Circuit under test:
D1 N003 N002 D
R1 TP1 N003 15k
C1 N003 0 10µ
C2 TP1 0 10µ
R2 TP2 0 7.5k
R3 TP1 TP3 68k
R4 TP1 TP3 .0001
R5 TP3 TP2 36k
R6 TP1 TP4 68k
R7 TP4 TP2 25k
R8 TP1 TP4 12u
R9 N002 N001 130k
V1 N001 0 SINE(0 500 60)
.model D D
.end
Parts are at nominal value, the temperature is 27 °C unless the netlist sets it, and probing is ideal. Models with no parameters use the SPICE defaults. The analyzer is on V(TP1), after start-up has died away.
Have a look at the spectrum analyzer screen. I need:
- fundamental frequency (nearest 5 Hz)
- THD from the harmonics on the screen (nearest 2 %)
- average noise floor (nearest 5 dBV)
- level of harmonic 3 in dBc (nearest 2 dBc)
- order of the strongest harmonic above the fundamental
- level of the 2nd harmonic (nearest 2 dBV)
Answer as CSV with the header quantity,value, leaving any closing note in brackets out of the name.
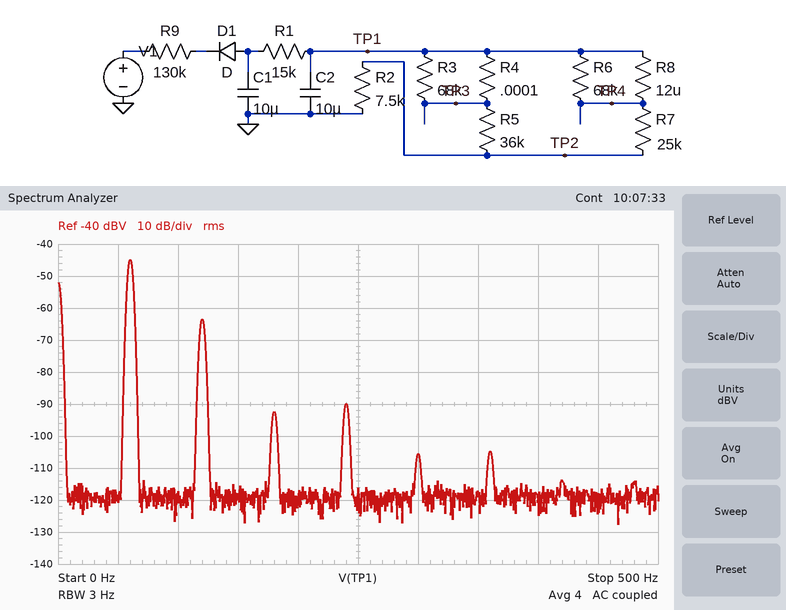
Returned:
quantity,value
fundamental frequency,60 Hz
THD from the harmonics on the screen,12 %
average noise floor,-120 dBV
level of harmonic 3 in dBc,-48 dBc
order of the strongest harmonic above the fundamental,2
level of the 2nd harmonic,-64 dBV
